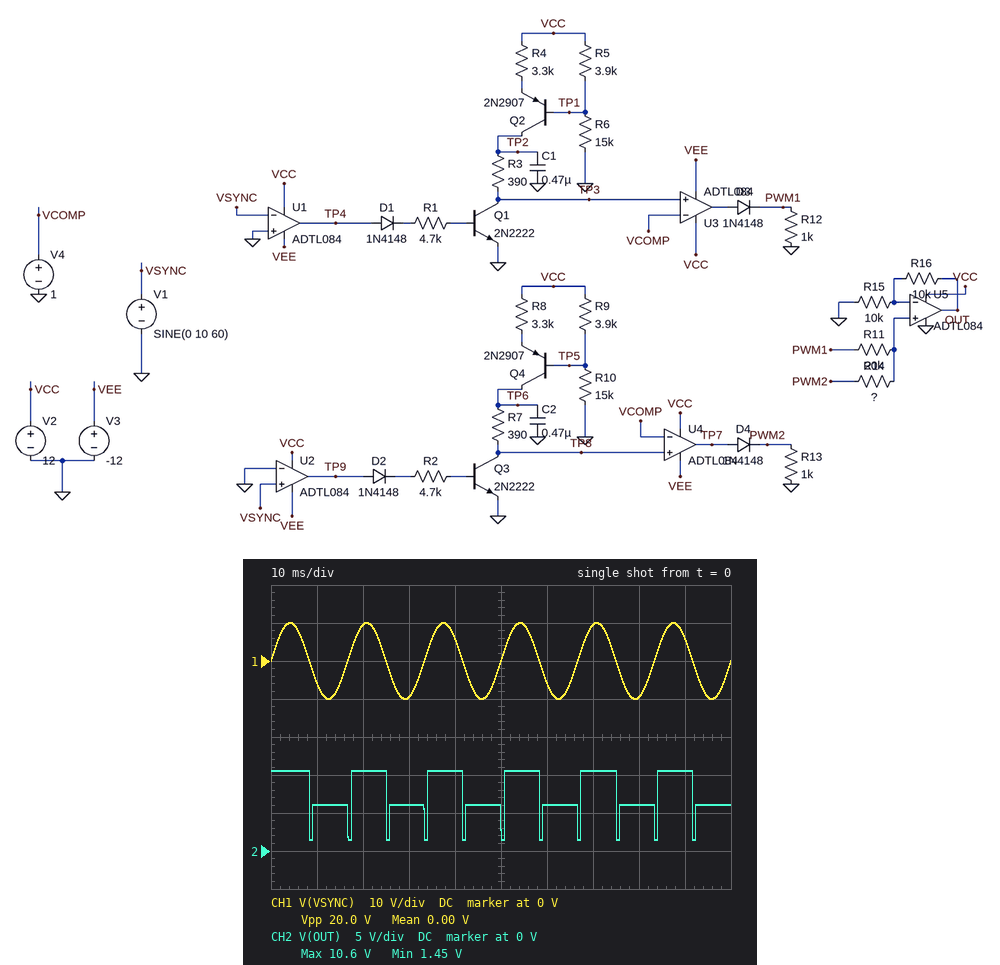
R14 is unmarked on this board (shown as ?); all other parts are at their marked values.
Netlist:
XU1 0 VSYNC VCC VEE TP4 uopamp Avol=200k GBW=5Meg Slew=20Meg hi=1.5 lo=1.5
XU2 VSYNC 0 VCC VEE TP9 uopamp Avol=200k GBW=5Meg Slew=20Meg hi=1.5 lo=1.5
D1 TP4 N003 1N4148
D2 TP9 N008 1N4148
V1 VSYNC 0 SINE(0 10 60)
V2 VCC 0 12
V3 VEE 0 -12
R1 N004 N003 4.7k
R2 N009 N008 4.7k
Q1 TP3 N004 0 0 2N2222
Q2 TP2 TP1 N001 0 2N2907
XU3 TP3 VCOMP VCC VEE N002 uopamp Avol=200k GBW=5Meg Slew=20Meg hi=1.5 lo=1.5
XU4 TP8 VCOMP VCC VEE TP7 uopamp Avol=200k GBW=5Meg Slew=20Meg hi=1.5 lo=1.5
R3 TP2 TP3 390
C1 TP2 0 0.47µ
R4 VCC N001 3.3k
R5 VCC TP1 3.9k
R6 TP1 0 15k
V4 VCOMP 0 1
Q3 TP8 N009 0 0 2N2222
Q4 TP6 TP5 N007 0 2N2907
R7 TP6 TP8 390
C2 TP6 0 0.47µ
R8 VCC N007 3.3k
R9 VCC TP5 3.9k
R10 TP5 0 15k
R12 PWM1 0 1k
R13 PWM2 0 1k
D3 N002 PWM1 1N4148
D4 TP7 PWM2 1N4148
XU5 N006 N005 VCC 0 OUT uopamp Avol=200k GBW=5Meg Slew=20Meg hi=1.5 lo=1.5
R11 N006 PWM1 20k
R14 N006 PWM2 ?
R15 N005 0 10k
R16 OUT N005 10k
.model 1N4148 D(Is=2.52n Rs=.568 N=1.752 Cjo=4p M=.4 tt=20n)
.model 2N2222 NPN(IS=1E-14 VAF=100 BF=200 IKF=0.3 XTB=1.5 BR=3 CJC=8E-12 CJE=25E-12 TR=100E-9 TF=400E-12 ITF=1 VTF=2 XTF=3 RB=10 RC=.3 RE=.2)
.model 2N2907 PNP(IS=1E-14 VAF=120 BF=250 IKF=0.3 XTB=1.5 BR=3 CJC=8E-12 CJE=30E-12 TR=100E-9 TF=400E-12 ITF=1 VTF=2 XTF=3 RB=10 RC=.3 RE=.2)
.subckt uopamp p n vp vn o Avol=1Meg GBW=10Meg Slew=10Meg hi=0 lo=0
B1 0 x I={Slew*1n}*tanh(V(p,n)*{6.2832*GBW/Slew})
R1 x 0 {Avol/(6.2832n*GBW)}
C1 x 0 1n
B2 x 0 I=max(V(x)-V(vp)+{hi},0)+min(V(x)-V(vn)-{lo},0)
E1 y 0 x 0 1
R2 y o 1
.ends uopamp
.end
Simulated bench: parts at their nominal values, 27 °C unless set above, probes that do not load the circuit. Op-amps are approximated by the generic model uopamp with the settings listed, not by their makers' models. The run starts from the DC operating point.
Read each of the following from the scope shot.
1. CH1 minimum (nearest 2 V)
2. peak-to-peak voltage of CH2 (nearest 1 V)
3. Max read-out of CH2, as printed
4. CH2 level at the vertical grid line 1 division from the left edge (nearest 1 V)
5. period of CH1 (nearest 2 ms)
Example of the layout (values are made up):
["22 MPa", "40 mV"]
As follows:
["-10 V", "9 V", "10.6 V", "6 V", "16 ms"]
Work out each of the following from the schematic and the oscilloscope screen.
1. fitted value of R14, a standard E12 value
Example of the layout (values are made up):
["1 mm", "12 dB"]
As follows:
["47 kΩ"]
